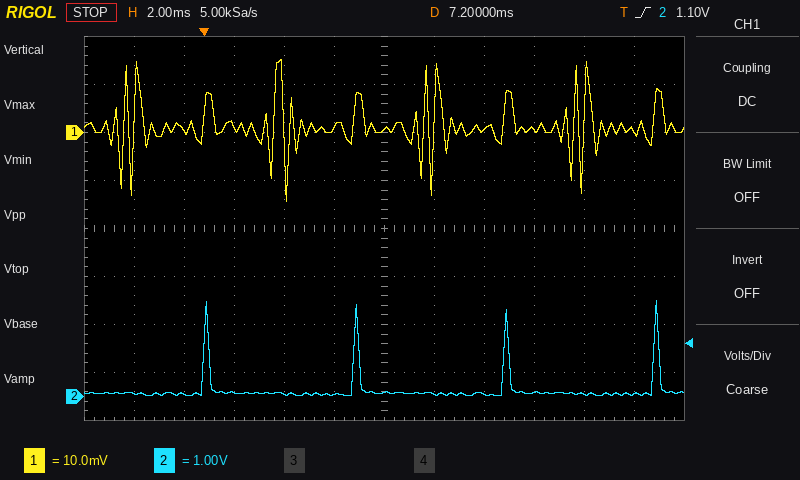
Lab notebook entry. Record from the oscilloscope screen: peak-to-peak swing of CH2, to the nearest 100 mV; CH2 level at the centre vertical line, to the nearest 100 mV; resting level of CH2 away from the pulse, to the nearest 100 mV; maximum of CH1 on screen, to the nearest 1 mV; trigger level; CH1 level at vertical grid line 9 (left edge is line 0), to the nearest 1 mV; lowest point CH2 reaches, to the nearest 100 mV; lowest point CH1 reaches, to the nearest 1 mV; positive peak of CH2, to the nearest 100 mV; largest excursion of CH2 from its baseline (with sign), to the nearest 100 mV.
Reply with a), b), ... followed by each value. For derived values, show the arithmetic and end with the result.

a) 2.0 V − (0.0 V) = 2.0 V
b) 100 mV
c) 100 mV
d) 15 mV
e) 1.10 V
f) 1 mV
g) 0.0 V
h) -14 mV
i) 2.0 V
j) 2.0 V − (100 mV) = +1.9 V
